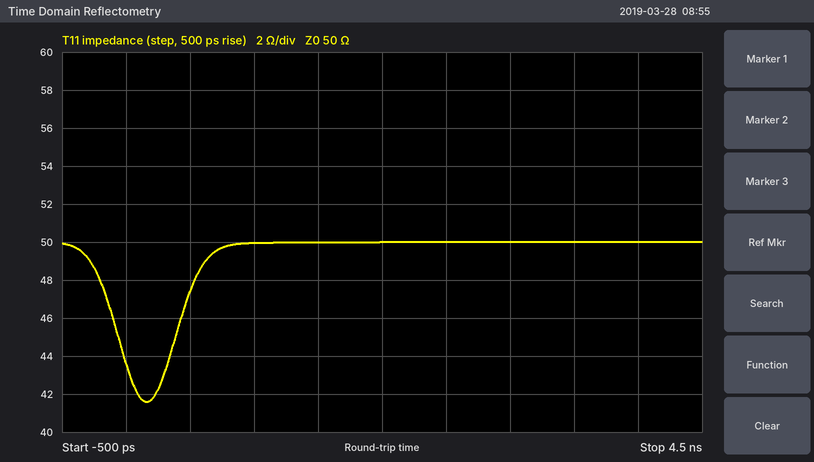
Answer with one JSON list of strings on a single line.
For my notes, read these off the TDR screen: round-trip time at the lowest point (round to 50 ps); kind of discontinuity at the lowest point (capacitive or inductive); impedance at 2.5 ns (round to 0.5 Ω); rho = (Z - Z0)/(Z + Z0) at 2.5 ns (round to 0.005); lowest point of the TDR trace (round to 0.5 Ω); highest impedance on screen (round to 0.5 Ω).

["150 ps", "capacitive", "50.0 Ω", "0.000", "41.5 Ω", "50.0 Ω"]
